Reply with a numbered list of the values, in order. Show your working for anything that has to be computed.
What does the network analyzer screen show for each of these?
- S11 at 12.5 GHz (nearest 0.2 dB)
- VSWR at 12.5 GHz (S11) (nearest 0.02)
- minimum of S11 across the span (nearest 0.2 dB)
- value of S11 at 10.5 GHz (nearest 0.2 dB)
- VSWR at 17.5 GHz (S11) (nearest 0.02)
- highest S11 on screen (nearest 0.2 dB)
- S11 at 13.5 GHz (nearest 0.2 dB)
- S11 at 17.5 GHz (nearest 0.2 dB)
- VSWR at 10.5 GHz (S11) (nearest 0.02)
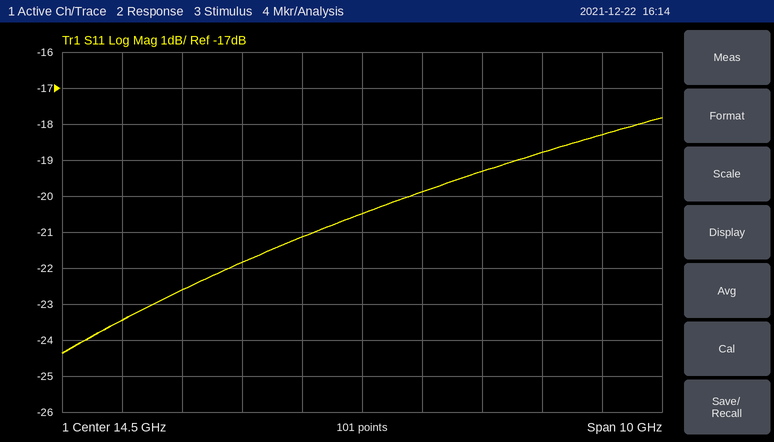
1. -21.8 dB
2. |Γ| = 10^(-21.8/20) = 0.0813; VSWR = (1 + 0.0813)/(1 − 0.0813) ≈ 1.18
3. -24.4 dB
4. -23.4 dB
5. |Γ| = 10^(-18.8/20) = 0.1148; VSWR = (1 + 0.1148)/(1 − 0.1148) ≈ 1.26
6. -17.8 dB
7. -21.2 dB
8. -18.8 dB
9. |Γ| = 10^(-23.4/20) = 0.0676; VSWR = (1 + 0.0676)/(1 − 0.0676) ≈ 1.15, so 1.14 to the nearest 0.02
